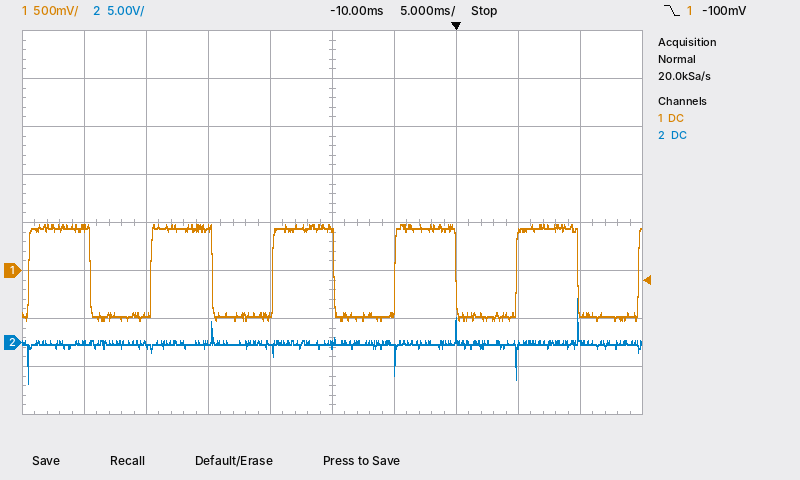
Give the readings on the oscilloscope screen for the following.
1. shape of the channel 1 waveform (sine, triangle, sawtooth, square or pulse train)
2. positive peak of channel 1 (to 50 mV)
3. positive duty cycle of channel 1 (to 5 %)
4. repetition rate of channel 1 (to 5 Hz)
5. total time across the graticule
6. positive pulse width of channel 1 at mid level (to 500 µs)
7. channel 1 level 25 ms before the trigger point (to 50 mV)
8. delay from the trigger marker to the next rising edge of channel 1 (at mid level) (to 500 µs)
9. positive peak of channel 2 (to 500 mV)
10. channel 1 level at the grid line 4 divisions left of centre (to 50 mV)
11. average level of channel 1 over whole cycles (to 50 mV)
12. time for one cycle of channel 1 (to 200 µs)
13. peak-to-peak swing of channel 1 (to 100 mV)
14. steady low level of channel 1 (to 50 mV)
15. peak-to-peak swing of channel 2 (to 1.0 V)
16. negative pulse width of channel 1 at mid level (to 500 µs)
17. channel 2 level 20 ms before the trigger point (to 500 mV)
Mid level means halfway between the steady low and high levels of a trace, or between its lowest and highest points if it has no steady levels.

square
500 mV
50 %
100 Hz
50 ms
5.0 ms
-450 mV
5.0 ms
4.5 V
450 mV
0 mV
9.8 ms
1.00 V
-500 mV
9.0 V
5.0 ms
0.0 V
